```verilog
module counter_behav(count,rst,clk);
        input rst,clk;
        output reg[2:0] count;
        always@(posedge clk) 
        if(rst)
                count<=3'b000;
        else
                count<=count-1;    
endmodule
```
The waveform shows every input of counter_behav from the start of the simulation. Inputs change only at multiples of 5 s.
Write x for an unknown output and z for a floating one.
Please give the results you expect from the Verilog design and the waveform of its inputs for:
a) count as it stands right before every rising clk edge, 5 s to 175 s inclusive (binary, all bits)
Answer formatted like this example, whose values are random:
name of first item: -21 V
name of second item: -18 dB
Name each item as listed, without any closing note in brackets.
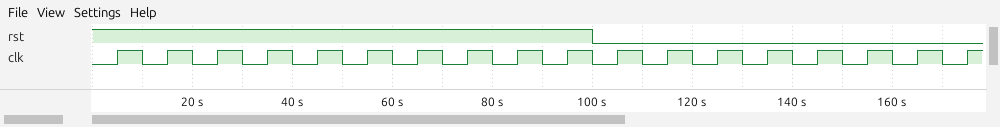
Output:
count as it stands right before every rising clk edge, 5 s to 175 s inclusive: x, 000, 000, 000, 000, 000, 000, 000, 000, 000, 000, 111, 110, 101, 100, 011, 010, 001
